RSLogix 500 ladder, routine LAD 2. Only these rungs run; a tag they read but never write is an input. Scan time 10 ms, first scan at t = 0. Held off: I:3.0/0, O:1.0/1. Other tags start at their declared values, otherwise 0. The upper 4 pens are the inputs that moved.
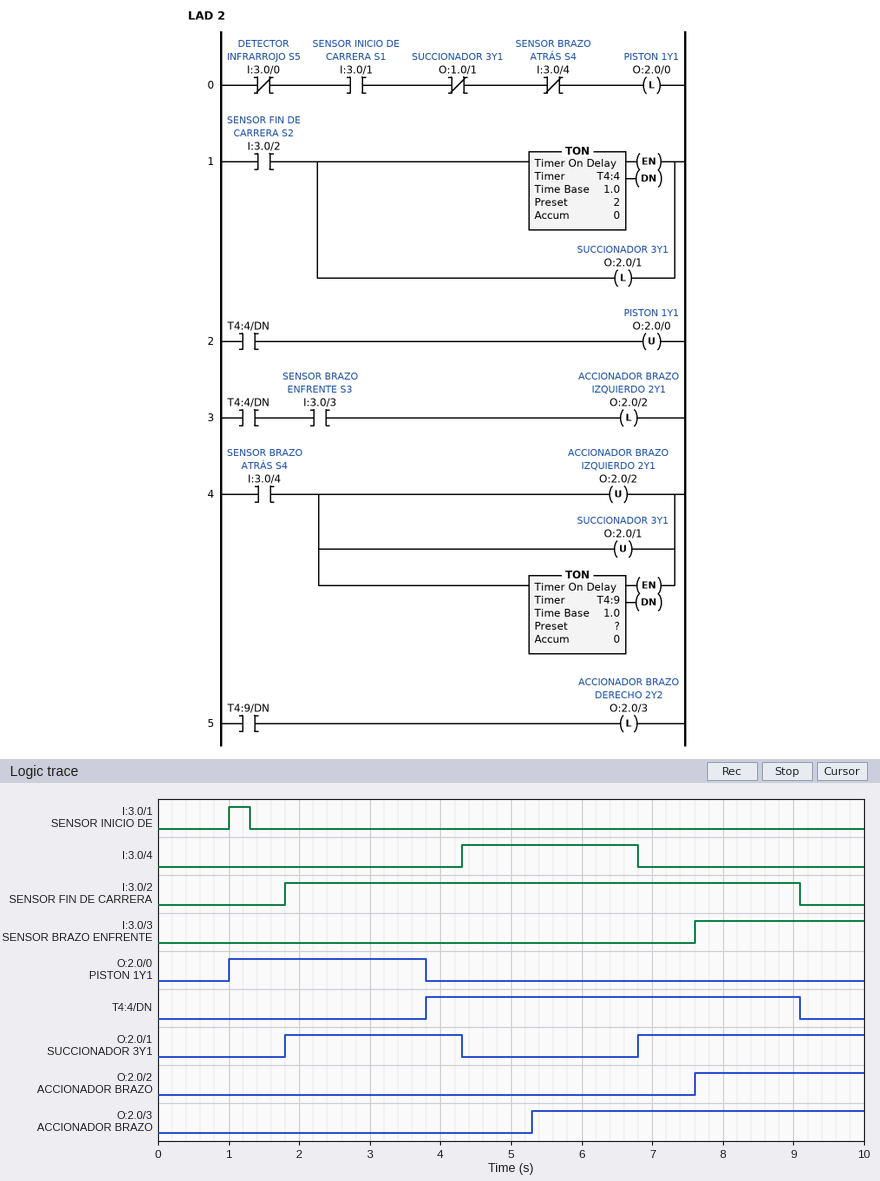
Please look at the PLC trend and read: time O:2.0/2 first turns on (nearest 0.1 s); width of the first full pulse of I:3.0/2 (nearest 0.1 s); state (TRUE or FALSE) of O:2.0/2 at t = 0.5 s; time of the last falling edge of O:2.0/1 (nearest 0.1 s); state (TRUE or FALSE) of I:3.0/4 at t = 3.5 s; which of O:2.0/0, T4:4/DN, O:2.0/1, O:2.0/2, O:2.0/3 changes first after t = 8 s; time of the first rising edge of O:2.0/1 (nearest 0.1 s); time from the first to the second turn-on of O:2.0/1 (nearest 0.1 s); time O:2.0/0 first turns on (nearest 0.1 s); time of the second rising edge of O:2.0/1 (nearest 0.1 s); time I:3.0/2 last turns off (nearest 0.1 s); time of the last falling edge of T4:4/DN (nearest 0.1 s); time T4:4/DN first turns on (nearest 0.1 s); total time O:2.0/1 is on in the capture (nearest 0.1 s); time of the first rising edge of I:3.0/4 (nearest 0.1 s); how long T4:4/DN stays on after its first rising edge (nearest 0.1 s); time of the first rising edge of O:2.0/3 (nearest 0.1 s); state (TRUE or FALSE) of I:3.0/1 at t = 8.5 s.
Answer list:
7.6 s
7.3 s
FALSE
4.3 s
FALSE
T4:4/DN
1.8 s
5.0 s
1.0 s
6.8 s
9.1 s
9.1 s
3.8 s
5.7 s
4.3 s
5.3 s
5.3 s
FALSE
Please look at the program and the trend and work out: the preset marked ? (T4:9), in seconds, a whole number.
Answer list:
1 s
